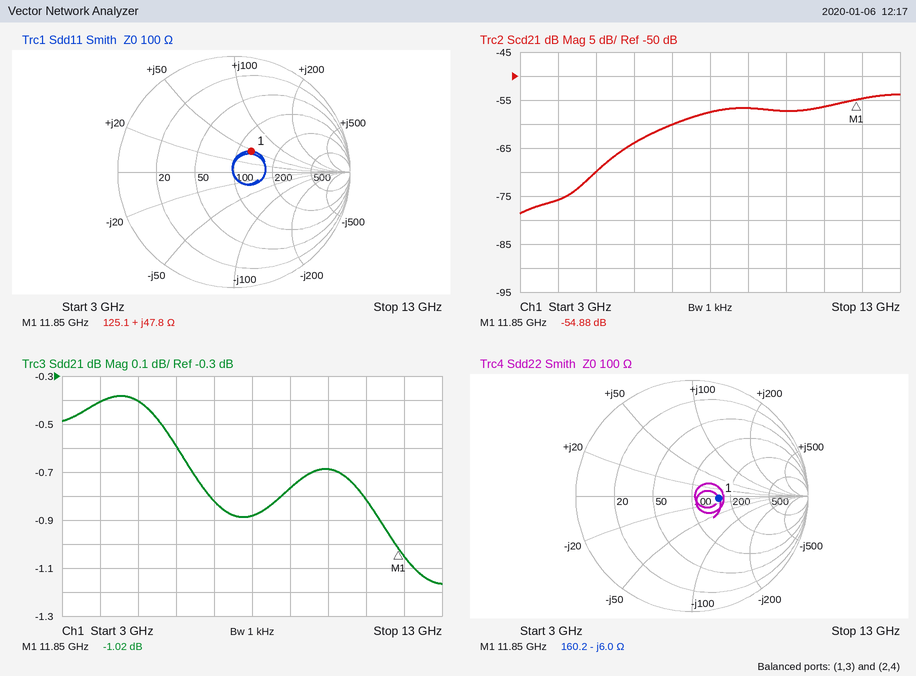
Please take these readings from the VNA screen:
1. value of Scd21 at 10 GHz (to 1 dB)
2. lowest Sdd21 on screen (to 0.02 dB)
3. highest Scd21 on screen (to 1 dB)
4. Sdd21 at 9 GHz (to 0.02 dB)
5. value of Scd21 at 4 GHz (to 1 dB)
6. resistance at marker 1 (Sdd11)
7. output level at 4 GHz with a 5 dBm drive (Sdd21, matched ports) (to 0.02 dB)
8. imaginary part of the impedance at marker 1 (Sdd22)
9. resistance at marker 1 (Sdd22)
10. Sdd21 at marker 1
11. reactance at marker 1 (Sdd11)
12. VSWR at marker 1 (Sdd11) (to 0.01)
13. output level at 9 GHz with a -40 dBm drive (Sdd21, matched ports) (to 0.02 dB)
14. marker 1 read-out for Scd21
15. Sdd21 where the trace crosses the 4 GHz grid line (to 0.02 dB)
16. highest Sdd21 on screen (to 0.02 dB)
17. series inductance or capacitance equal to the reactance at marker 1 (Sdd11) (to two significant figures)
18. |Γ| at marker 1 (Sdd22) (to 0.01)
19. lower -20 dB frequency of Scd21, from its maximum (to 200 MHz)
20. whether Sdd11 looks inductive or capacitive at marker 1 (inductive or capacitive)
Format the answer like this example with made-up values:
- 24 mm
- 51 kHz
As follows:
- -57 dB
- -1.16 dB
- -54 dB
- -0.76 dB
- -76 dB
- 125.1 Ω
- 4.60 dBm
- -6.0 Ω
- 160.2 Ω
- -1.02 dB
- +47.8 Ω
- 1.61
- -40.76 dBm
- -54.88 dB
- -0.40 dB
- -0.38 dB
- 640 pH
- 0.23
- 4.4 GHz
- inductive
